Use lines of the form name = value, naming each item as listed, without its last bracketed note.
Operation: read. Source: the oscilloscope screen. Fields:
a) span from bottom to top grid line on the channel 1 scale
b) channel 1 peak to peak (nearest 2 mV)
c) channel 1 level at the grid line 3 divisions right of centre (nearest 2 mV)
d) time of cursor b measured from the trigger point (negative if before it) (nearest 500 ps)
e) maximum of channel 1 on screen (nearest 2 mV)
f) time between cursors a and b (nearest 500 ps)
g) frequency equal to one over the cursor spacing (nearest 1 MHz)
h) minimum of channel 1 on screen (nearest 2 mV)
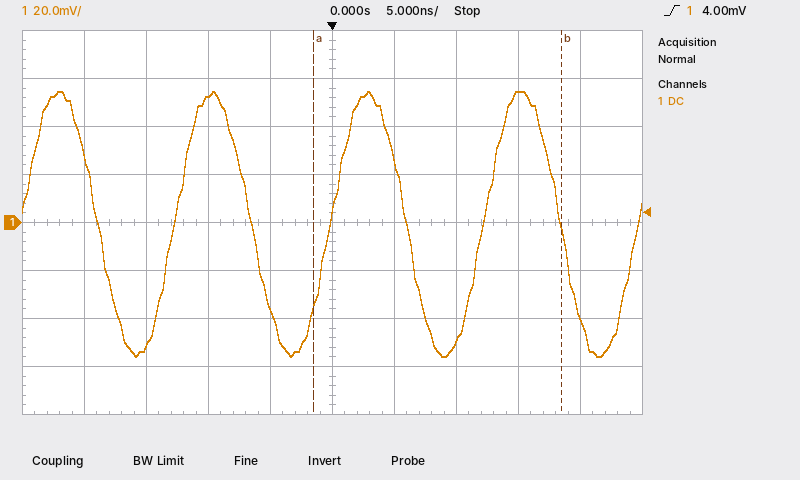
span from bottom to top grid line on the channel 1 scale = 160 mV
channel 1 peak to peak = 110 mV
channel 1 level at the grid line 3 divisions right of centre = 54 mV
time of cursor b measured from the trigger point (negative if before it) = +18.5 ns
maximum of channel 1 on screen = 54 mV
time between cursors a and b = 20.0 ns
frequency equal to one over the cursor spacing = 50 MHz
minimum of channel 1 on screen = -56 mV
